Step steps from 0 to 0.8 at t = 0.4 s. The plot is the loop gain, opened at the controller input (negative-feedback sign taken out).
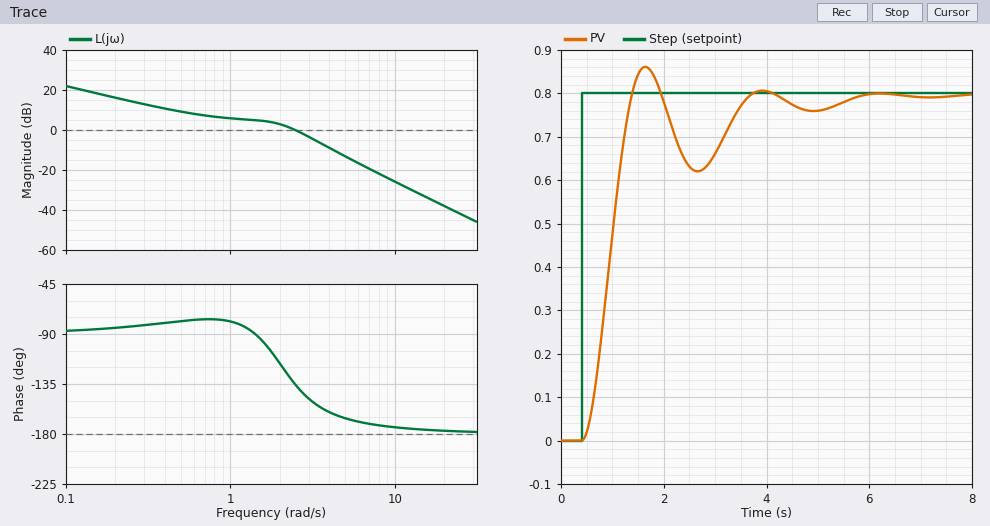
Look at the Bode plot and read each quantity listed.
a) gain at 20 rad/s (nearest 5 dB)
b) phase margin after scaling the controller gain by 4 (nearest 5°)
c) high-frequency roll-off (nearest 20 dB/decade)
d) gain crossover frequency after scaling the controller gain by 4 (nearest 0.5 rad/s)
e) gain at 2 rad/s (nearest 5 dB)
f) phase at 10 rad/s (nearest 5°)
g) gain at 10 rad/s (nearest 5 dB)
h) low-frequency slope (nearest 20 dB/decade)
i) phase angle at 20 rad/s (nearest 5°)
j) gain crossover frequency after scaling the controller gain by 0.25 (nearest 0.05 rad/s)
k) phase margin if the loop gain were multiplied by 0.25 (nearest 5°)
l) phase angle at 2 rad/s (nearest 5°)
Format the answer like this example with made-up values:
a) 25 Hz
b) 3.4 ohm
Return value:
a) -40 dB
b) 15°
c) -40 dB/decade
d) 4.5 rad/s
e) 5 dB
f) -175°
g) -25 dB
h) -20 dB/decade
i) -175°
j) 0.35 rad/s
k) 100°
l) -115°
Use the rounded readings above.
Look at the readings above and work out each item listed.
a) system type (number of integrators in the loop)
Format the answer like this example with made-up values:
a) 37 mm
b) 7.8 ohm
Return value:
a) 1
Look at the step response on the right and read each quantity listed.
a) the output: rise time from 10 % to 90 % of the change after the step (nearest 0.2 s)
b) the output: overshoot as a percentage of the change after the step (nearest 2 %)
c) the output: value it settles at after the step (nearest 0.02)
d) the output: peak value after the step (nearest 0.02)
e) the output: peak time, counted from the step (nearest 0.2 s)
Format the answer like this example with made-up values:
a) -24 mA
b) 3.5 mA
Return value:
a) 0.6 s
b) 8 %
c) 0.80
d) 0.86
e) 1.2 s
